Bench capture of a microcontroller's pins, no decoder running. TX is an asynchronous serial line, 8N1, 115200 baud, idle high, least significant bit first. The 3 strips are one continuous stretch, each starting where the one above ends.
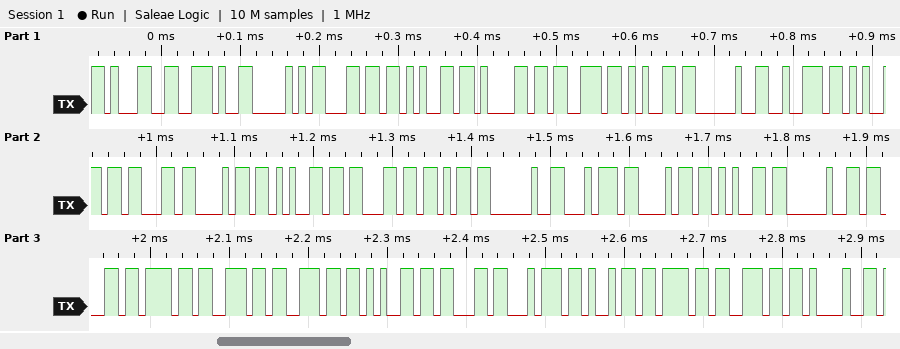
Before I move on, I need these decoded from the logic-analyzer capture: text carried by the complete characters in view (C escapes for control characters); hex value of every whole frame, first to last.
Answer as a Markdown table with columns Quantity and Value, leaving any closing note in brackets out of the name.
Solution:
| Quantity | Value |
|---|---|
| text carried by the complete characters in view | "1.Please recheck the connection!" |
| hex value of every whole frame, first to last | 0x31 0x2E 0x50 0x6C 0x65 0x61 0x73 0x65 0x20 0x72 0x65 0x63 0x68 0x65 0x63 0x6B 0x20 0x74 0x68 0x65 0x20 0x63 0x6F 0x6E 0x6E 0x65 0x63 0x74 0x69 0x6F 0x6E 0x21 |
